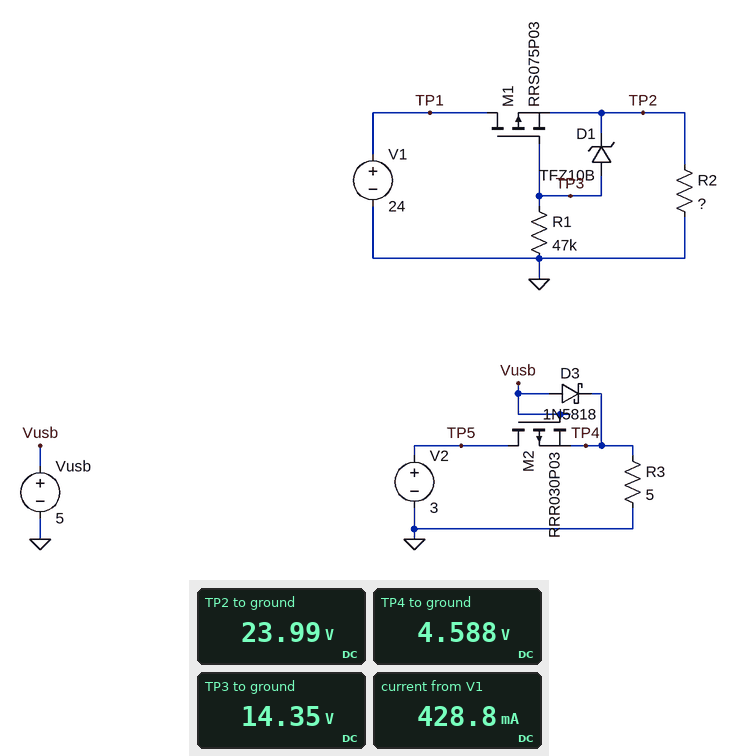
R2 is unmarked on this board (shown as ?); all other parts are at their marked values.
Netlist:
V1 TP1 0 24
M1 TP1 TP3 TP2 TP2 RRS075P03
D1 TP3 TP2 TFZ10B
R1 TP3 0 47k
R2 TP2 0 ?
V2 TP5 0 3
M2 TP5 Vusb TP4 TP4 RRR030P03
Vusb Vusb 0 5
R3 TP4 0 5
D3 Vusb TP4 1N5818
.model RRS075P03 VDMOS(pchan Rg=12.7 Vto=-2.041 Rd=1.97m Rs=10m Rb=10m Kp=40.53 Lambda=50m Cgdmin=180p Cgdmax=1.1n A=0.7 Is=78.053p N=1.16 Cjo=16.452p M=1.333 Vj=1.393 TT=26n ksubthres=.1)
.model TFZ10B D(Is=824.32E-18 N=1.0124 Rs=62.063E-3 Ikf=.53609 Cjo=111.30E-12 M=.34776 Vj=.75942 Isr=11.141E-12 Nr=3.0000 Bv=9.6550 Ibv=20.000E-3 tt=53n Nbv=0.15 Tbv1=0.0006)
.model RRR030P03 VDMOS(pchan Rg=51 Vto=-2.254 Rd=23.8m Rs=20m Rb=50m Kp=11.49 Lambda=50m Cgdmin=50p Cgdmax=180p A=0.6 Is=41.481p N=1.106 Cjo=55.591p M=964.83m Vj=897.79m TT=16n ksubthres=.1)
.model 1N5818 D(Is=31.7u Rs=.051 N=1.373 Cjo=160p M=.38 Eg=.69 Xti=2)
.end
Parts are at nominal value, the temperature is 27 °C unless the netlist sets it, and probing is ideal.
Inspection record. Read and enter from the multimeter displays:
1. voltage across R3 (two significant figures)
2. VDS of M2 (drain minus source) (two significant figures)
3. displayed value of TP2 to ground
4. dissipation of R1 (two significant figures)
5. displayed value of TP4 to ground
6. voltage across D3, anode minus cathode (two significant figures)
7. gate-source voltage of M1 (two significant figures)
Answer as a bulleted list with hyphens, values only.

- 4.6 V
- -1.6 V
- 23.99 V
- 4.4 mW
- 4.588 V
- 410 mV
- -9.6 V
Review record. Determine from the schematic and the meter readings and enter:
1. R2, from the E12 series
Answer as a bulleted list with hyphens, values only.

- 56 Ω
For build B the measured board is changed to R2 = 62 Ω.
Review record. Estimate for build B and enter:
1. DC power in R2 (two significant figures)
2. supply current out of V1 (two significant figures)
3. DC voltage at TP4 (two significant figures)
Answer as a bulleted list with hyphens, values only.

- 9.3 W
- 390 mA
- 4.6 V
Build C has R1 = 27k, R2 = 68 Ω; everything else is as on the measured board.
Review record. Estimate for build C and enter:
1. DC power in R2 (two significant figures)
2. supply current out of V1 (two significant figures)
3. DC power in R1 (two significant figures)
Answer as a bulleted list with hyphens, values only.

- 8.5 W
- 350 mA
- 7.6 mW
